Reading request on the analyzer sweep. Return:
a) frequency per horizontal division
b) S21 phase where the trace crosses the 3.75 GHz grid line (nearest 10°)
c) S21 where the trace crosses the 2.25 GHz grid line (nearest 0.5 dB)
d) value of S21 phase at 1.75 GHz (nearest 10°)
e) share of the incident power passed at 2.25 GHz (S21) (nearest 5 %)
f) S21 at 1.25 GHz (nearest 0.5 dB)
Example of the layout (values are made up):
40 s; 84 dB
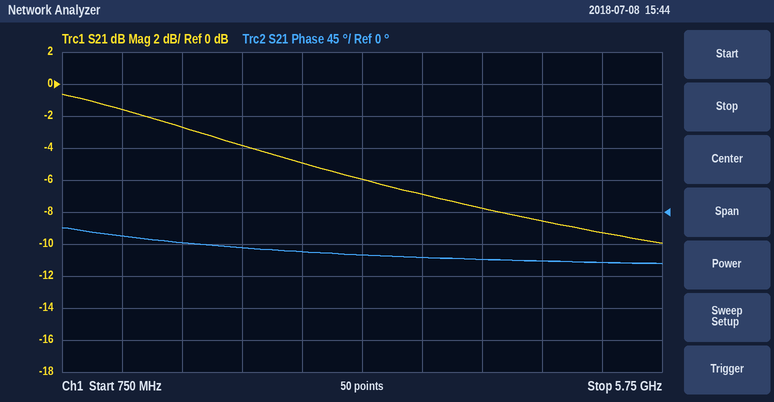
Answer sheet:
500 MHz; -60°; -4.0 dB; -40°; 40 %; -1.5 dB
